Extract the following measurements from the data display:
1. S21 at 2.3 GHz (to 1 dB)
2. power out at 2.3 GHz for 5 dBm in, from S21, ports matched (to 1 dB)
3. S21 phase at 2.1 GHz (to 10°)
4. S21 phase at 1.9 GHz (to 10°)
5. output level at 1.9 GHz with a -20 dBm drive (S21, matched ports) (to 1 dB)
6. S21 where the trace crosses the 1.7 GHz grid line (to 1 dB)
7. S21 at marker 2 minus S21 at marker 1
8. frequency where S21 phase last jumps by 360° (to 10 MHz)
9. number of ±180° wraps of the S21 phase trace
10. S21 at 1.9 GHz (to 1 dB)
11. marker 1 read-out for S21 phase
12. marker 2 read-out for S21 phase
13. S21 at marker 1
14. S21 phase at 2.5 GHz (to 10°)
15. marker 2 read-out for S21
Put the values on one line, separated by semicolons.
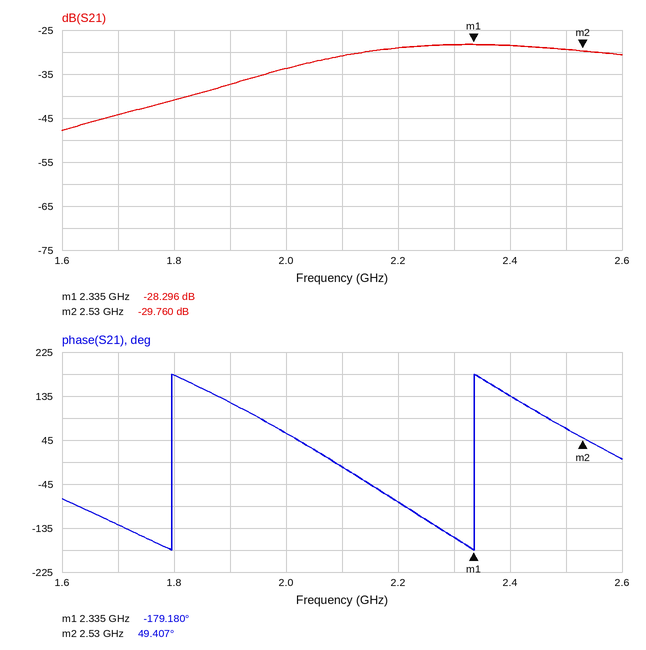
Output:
-28 dB; -23 dBm; -10°; 120°; -57 dBm; -44 dB; -1.464 dB; 2.34 GHz; 2; -37 dB; -179.180°; 49.407°; -28.296 dB; 70°; -29.760 dB
